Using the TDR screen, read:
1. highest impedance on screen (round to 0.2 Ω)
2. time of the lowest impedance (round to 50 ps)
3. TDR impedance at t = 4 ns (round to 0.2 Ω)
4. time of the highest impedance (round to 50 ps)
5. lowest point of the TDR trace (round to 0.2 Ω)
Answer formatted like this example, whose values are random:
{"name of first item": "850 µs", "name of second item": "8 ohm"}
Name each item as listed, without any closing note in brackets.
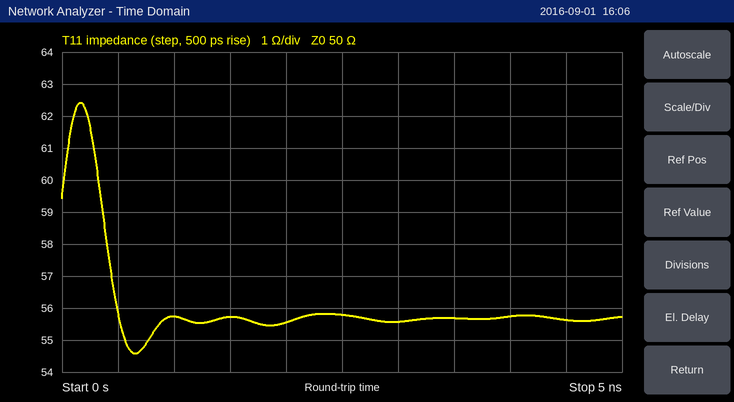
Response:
{"highest impedance on screen": "62.4 Ω", "time of the lowest impedance": "650 ps", "TDR impedance at t = 4 ns": "55.8 Ω", "time of the highest impedance": "150 ps", "lowest point of the TDR trace": "54.6 Ω"}
